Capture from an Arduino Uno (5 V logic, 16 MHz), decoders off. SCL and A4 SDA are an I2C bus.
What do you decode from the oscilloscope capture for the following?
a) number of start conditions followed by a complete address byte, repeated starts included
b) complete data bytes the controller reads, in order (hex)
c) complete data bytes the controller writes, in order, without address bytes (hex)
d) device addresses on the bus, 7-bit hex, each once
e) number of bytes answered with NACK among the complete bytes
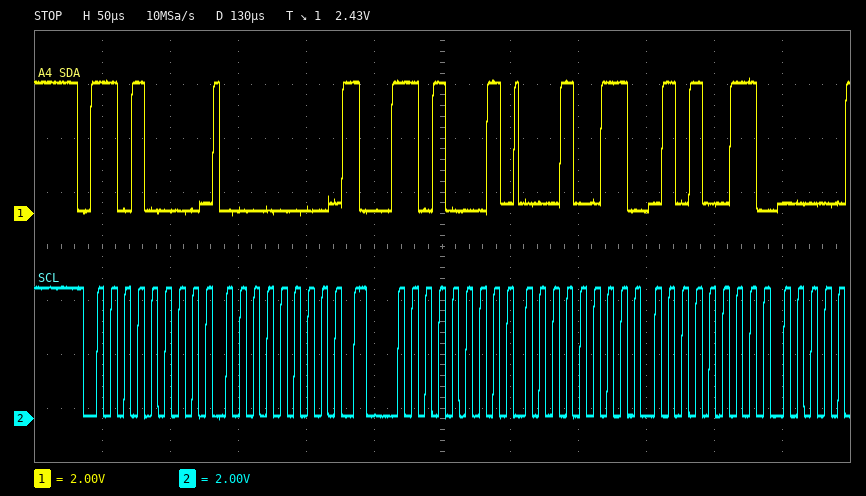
2
13 53
00
0x68
0
